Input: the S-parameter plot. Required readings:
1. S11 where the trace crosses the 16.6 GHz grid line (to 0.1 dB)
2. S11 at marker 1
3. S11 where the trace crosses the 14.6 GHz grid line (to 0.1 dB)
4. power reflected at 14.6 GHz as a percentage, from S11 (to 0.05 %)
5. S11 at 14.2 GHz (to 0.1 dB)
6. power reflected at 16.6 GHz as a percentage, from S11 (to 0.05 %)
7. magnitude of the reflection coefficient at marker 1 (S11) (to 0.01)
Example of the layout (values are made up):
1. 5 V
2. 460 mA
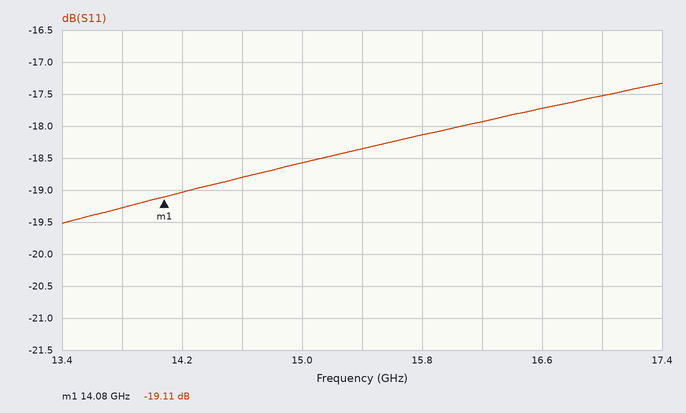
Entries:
1. -17.7 dB
2. -19.11 dB
3. -18.8 dB
4. 1.30 %
5. -19.0 dB
6. 1.70 %
7. 0.11
